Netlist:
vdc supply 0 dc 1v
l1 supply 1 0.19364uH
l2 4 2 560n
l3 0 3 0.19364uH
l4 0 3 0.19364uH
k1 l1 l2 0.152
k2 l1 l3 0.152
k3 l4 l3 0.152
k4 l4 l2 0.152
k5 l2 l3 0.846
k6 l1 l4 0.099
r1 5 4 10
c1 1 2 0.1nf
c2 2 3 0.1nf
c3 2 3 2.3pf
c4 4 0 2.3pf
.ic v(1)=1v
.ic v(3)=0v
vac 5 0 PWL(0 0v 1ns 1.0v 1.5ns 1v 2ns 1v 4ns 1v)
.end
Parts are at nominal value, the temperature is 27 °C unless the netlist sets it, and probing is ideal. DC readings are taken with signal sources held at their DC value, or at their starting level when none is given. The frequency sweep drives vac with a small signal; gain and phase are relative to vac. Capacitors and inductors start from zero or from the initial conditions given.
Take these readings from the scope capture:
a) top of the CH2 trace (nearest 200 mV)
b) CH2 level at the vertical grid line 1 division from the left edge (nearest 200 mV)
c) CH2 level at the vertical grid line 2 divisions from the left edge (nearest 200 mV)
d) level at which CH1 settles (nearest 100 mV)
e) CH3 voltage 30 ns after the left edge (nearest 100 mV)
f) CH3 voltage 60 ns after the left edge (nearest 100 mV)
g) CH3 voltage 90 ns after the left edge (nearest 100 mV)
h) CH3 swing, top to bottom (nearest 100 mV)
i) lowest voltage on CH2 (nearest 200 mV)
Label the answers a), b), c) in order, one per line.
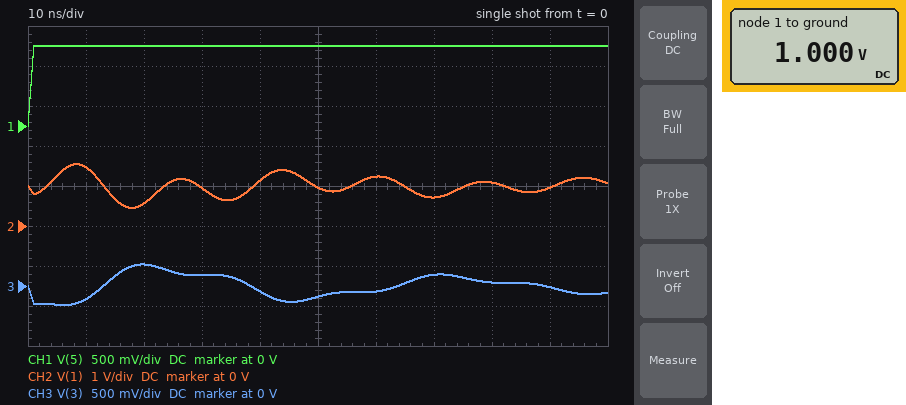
a) 1.6 V
b) 1.4 V
c) 600 mV
d) 1.0 V
e) 100 mV
f) -100 mV
g) 0 V
h) 500 mV
i) 400 mV
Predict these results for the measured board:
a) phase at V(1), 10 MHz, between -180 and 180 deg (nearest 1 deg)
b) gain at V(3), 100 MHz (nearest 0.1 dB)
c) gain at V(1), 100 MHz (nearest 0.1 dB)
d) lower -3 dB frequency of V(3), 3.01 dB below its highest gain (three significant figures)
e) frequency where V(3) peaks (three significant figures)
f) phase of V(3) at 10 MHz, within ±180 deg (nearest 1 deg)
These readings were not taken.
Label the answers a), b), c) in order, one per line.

a) 171 deg
b) -14.2 dB
c) -6.6 dB
d) 18.5 MHz
e) 20.6 MHz
f) -9 deg
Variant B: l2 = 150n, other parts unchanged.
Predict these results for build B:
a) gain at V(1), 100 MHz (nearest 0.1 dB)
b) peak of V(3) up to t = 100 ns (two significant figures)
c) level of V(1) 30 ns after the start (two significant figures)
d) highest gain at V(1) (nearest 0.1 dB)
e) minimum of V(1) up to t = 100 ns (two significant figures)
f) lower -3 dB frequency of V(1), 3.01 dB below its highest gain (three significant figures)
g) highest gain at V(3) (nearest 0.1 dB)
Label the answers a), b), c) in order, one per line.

a) -24.1 dB
b) 390 mV
c) 1.3 V
d) 10.1 dB
e) 330 mV
f) 29.2 MHz
g) 4.9 dB
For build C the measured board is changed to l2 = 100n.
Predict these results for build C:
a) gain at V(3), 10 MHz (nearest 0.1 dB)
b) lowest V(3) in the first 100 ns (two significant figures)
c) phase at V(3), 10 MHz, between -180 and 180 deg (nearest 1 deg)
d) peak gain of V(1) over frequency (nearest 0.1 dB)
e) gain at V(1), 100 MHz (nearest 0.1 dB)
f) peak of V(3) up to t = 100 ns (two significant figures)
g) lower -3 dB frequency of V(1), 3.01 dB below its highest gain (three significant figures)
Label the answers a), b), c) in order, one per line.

a) -52.9 dB
b) -570 mV
c) -8 deg
d) 11.5 dB
e) -4.1 dB
f) 640 mV
g) 31.3 MHz
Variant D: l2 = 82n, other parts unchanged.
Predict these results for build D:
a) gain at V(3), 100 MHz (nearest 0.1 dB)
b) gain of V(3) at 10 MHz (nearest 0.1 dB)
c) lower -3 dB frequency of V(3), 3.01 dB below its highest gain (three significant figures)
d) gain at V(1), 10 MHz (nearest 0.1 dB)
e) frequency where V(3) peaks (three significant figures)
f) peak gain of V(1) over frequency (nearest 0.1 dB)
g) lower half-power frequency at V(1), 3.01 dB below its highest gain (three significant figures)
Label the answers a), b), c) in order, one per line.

a) 4.8 dB
b) -49.6 dB
c) 59.7 MHz
d) -22.0 dB
e) 75.1 MHz
f) 12.0 dB
g) 32.1 MHz
